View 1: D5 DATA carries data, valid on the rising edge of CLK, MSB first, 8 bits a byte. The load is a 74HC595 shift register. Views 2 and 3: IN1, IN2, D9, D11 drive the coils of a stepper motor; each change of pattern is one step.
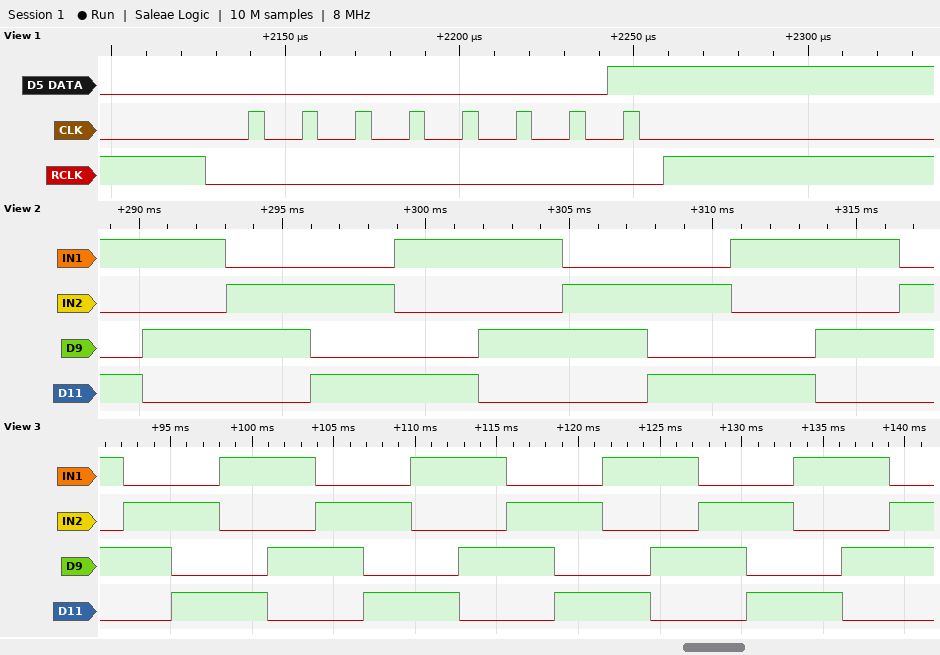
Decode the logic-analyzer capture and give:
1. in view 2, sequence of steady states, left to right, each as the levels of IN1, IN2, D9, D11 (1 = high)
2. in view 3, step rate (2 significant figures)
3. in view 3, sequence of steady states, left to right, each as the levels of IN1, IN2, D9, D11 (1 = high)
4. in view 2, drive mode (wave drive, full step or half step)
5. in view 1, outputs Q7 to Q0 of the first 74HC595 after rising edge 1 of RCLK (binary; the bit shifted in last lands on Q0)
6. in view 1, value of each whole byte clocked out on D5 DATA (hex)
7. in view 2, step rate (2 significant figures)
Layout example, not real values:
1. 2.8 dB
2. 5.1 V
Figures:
1. 1001 1010 0110 0101 1001 1010 0110 0101 1001 1010 0110
2. 340 steps/s
3. 1010 0110 0101 1001 1010 0110 0101 1001 1010 0110 0101 1001 1010 0110 0101 1001 1010 0110
4. full step
5. 00000001
6. 01
7. 340 steps/s
